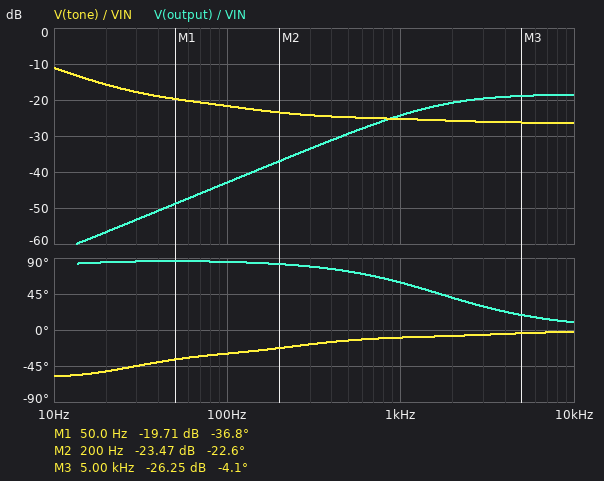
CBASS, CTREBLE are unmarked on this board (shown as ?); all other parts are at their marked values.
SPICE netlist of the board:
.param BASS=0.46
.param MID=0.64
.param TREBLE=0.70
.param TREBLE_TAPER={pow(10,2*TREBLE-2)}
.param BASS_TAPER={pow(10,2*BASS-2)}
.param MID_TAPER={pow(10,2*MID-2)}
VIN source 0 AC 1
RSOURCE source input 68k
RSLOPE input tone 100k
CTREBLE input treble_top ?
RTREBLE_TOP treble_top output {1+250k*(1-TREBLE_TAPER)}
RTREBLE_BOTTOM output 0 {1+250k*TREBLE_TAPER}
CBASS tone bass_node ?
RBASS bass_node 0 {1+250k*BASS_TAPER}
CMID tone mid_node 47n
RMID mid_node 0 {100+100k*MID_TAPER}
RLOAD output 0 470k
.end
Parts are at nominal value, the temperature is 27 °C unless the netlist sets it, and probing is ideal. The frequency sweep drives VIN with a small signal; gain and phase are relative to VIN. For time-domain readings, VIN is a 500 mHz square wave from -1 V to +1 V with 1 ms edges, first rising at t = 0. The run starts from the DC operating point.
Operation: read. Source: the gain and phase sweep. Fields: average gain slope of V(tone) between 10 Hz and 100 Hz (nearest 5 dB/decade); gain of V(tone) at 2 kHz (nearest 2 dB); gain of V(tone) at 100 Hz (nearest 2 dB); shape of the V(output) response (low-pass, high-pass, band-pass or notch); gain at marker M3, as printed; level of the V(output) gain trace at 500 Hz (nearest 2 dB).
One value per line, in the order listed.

-10 dB/decade
-26 dB
-22 dB
high-pass
-26.25 dB
-30 dB
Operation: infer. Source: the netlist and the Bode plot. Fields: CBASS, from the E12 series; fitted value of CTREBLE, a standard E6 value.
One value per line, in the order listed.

270 nF
330 pF
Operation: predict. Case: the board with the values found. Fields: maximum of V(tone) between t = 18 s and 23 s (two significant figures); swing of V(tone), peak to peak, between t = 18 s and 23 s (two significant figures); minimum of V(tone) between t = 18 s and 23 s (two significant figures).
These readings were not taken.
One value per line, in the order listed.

1.0 V
2.0 V
-1.0 V
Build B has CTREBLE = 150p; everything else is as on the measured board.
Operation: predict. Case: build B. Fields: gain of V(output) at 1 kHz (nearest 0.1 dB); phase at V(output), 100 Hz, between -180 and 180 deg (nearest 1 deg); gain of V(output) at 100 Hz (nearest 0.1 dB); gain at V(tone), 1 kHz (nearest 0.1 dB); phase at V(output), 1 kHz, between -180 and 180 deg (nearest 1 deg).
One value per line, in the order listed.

-30.1 dB
87 deg
-49.7 dB
-25.0 dB
75 deg
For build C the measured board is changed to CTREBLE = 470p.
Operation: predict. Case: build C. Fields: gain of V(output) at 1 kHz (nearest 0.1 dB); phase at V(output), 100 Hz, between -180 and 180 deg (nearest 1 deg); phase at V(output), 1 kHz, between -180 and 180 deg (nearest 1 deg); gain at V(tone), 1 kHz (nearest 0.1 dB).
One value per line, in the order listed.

-22.2 dB
84 deg
50 deg
-25.5 dB
